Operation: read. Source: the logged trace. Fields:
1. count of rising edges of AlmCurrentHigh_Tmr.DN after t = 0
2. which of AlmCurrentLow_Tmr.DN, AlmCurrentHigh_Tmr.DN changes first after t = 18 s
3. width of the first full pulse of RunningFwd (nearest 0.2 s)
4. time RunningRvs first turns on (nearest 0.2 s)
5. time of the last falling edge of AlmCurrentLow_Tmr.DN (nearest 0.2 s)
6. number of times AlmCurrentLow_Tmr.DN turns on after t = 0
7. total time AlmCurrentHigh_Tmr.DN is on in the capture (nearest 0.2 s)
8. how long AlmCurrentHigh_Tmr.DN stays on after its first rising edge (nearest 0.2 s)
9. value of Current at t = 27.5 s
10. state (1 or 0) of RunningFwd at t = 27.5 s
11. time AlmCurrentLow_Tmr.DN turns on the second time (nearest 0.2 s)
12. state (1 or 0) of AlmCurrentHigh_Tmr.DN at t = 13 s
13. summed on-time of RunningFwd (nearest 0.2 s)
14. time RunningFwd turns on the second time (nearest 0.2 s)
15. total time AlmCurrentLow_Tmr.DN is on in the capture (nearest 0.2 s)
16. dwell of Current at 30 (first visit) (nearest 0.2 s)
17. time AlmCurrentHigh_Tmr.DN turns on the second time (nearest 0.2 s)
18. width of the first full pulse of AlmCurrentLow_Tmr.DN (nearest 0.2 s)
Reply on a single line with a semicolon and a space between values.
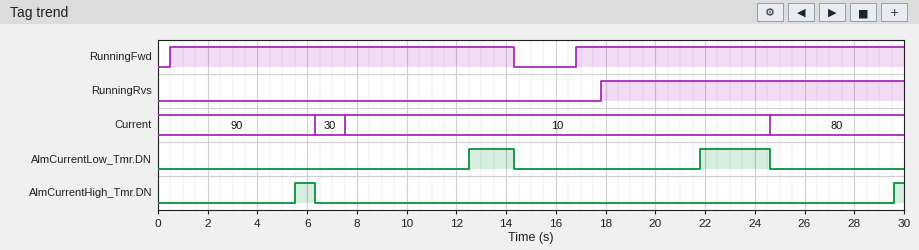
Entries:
2; AlmCurrentLow_Tmr.DN; 13.8 s; 17.8 s; 24.6 s; 2; 1.2 s; 0.8 s; 80; 1; 21.8 s; 0; 27.0 s; 16.8 s; 4.6 s; 1.2 s; 29.6 s; 1.8 s
